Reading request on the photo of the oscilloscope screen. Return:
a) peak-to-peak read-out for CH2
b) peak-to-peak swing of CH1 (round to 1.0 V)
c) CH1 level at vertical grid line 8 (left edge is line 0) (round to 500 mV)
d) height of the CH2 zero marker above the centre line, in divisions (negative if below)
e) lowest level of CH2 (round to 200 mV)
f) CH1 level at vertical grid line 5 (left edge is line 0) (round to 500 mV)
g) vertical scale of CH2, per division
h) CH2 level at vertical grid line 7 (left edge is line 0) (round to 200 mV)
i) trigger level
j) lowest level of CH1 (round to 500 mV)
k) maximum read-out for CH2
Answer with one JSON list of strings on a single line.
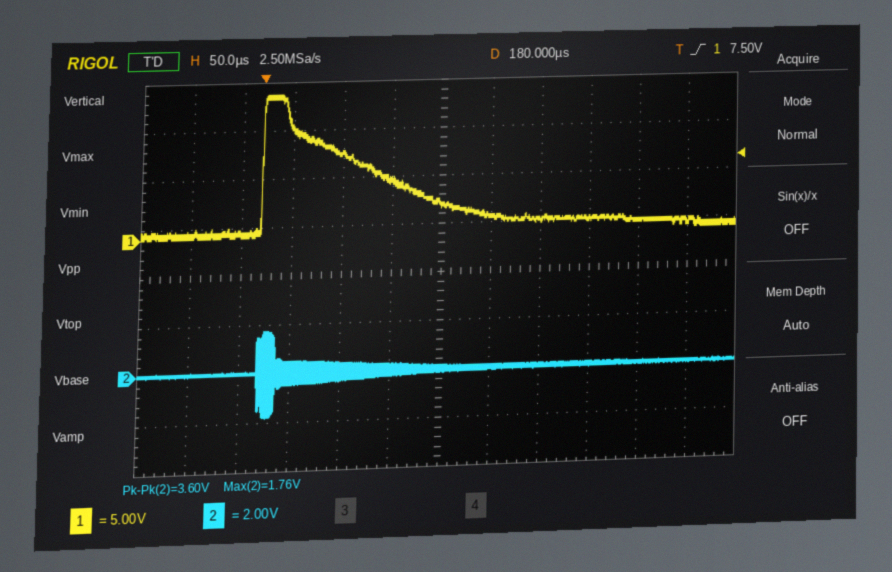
["3.60 V", "15.0 V", "1.0 V", "-2.0 div", "-1.8 V", "5.5 V", "2 V", "0.0 V", "7.50 V", "0.0 V", "1.76 V"]
